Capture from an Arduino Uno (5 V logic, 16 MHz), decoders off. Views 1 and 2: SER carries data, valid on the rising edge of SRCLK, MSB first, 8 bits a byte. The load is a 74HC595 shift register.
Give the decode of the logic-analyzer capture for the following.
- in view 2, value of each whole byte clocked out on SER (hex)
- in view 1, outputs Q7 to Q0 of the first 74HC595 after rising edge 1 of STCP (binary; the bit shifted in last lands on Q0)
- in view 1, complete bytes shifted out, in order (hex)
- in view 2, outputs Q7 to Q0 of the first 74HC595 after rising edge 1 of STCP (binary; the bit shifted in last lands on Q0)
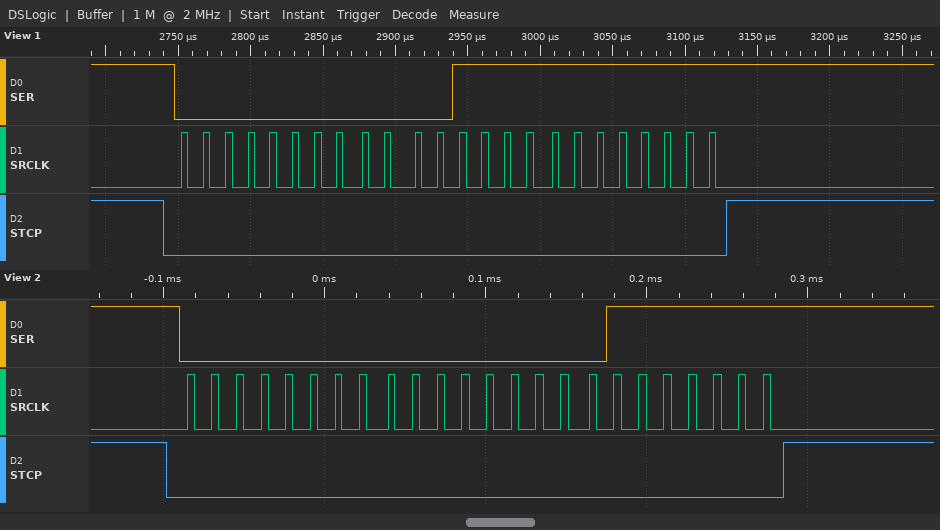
00 00 7F
11111111
00 0F FF
01111111
